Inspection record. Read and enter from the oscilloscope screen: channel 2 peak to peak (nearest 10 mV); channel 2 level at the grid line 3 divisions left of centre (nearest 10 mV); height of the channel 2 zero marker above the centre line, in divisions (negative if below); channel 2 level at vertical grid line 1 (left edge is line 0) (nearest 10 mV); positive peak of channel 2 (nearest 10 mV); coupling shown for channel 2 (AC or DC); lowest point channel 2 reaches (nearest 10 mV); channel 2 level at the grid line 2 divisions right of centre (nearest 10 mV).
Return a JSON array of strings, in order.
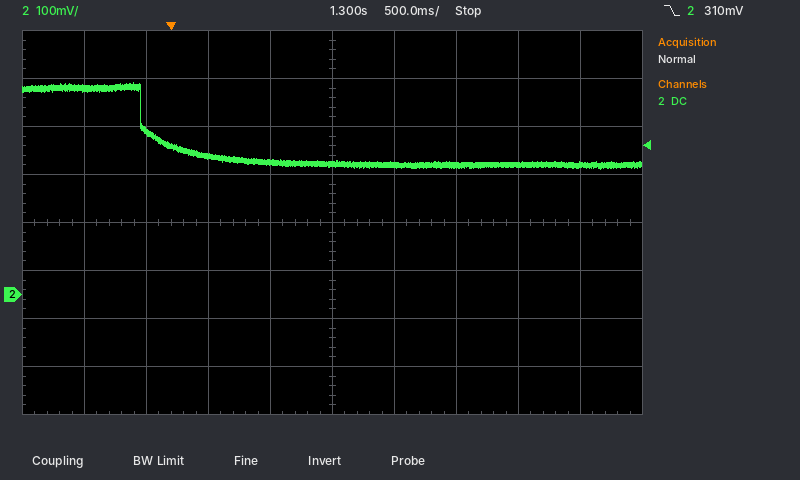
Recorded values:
["180 mV", "340 mV", "-1.5 div", "430 mV", "440 mV", "DC", "260 mV", "270 mV"]
